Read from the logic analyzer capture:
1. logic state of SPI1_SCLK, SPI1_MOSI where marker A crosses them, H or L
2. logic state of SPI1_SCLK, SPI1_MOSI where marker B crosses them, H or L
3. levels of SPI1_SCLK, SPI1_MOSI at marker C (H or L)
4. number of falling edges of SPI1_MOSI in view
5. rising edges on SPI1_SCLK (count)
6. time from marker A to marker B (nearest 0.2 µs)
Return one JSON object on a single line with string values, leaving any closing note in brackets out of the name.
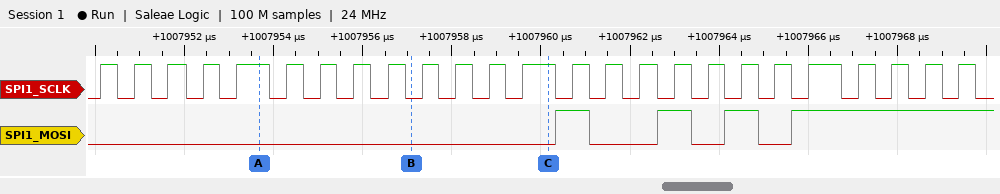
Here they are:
{"logic state of SPI1_SCLK, SPI1_MOSI where marker A crosses them, H or L": "SPI1_SCLK=H, SPI1_MOSI=L", "logic state of SPI1_SCLK, SPI1_MOSI where marker B crosses them, H or L": "SPI1_SCLK=L, SPI1_MOSI=L", "levels of SPI1_SCLK, SPI1_MOSI at marker C": "SPI1_SCLK=H, SPI1_MOSI=L", "number of falling edges of SPI1_MOSI in view": "3", "rising edges on SPI1_SCLK": "25", "time from marker A to marker B": "3.4 µs"}
